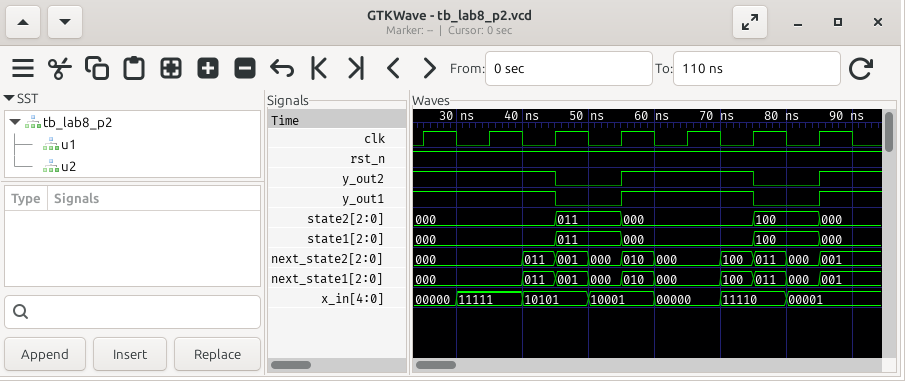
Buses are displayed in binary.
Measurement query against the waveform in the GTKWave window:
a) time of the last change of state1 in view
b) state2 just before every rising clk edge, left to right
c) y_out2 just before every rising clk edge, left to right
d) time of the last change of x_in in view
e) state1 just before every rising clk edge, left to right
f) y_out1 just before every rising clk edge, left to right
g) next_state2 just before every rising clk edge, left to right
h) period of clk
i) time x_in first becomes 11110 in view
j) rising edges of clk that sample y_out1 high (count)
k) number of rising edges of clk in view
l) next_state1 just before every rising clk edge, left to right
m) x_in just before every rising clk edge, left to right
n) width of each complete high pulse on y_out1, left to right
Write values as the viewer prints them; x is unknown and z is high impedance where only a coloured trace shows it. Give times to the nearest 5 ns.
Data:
85 ns
000, 000, 000, 011, 000, 000, 100
1 1 1 0 1 1 0
80 ns
000, 000, 000, 011, 000, 000, 100
1 1 1 0 1 1 0
000, 000, 011, 000, 000, 100, 000
10 ns
70 ns
5
7
000, 000, 011, 000, 000, 100, 000
00000, 11111, 10101, 10001, 00000, 11110, 00001
20 ns
